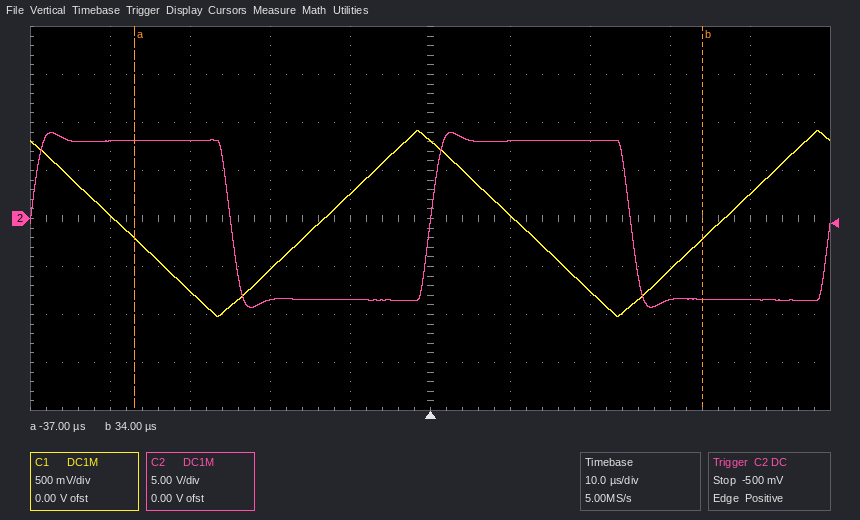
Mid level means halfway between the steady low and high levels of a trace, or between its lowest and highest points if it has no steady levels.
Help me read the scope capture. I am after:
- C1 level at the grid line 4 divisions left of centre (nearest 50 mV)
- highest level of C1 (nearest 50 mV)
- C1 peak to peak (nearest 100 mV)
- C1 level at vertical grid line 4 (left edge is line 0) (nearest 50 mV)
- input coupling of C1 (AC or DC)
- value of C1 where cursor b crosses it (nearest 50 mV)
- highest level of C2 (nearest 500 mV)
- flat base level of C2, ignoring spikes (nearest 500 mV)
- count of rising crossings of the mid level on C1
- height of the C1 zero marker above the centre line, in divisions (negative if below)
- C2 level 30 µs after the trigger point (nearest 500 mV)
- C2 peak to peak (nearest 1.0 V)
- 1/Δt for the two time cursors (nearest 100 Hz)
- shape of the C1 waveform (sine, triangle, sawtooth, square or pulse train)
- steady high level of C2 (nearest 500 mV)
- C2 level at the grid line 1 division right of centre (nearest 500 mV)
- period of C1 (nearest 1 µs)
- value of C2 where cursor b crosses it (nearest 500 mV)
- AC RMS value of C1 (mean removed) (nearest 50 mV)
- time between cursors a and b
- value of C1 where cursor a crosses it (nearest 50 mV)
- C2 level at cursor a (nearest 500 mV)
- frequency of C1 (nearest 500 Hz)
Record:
50 mV
900 mV
1.90 V
250 mV
DC
-200 mV
9.0 V
-8.5 V
2
0.0 div
-8.5 V
18.0 V
14.1 kHz
triangle
8.0 V
8.0 V
50 µs
-8.5 V
550 mV
71 µs
-200 mV
8.0 V
20.0 kHz
